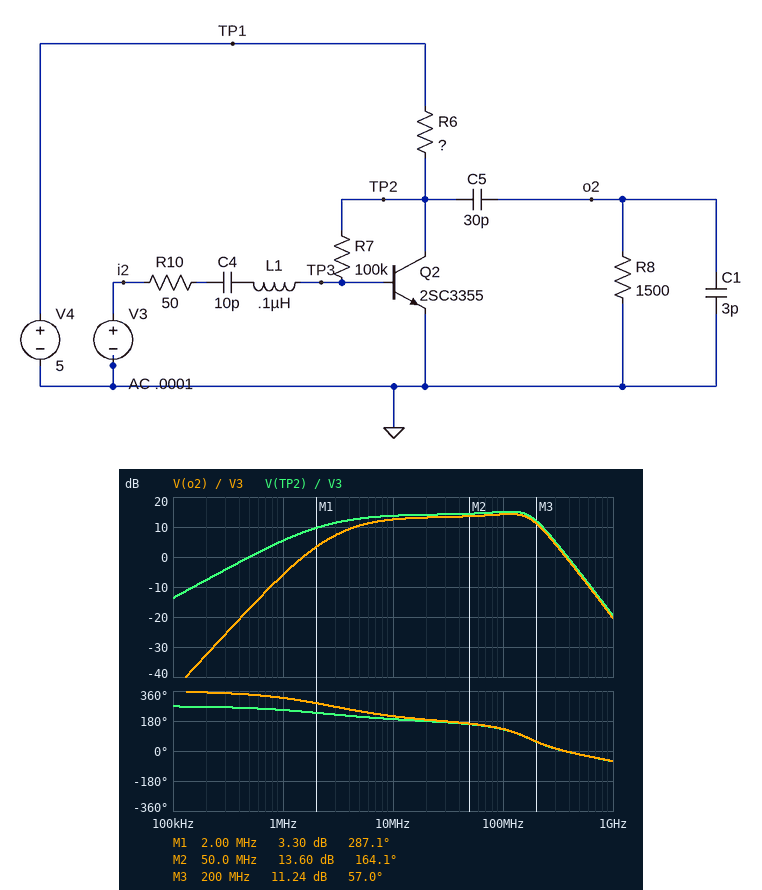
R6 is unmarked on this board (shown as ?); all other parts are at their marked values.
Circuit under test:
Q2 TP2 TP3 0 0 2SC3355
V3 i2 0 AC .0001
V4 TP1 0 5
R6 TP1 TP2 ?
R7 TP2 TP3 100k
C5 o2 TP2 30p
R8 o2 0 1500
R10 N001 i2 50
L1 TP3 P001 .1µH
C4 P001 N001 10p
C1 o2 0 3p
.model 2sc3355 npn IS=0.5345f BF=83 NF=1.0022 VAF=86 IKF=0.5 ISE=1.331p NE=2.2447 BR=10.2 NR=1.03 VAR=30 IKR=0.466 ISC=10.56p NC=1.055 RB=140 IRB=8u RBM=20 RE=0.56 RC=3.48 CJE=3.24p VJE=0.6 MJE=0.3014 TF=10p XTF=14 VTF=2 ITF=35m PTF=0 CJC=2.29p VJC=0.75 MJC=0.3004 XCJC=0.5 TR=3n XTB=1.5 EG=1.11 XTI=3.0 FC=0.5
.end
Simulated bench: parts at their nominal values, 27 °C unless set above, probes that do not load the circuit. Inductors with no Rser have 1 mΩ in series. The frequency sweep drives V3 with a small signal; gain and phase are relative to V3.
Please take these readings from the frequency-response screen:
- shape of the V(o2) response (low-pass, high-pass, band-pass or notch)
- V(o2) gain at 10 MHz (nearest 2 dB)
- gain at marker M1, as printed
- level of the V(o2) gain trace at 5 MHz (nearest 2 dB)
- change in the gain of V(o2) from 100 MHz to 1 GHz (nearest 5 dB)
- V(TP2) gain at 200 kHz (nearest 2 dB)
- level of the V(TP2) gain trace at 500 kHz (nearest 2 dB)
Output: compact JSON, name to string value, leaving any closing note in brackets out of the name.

{"shape of the V(o2) response": "band-pass", "V(o2) gain at 10 MHz": "12 dB", "gain at marker M1, as printed": "3.30 dB", "level of the V(o2) gain trace at 5 MHz": "10 dB", "change in the gain of V(o2) from 100 MHz to 1 GHz": "-35 dB", "V(TP2) gain at 200 kHz": "-8 dB", "level of the V(TP2) gain trace at 500 kHz": "0 dB"}
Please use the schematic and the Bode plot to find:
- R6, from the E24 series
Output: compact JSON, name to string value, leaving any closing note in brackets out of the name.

{"R6, from the E24 series": "620 Ω"}
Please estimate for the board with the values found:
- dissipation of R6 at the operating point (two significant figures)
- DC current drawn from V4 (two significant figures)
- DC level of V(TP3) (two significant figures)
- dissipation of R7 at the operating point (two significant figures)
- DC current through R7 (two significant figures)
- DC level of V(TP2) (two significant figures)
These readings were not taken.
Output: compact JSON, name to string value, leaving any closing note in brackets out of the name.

{"dissipation of R6 at the operating point": "3.3 mW", "DC current drawn from V4": "2.3 mA", "DC level of V(TP3)": "760 mV", "dissipation of R7 at the operating point": "79 µW", "DC current through R7": "28 µA", "DC level of V(TP2)": "3.6 V"}
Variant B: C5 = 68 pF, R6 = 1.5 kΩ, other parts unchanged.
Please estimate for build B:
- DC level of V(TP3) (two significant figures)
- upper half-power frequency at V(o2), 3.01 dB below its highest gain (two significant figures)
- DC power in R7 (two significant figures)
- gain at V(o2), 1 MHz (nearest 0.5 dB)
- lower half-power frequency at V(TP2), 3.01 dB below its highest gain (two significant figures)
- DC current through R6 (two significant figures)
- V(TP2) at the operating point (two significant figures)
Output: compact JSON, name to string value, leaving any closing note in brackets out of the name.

{"DC level of V(TP3)": "750 mV", "upper half-power frequency at V(o2), 3.01 dB below its highest gain": "190 MHz", "DC power in R7": "37 µW", "gain at V(o2), 1 MHz": "2.5 dB", "lower half-power frequency at V(TP2), 3.01 dB below its highest gain": "2.1 MHz", "DC current through R6": "1.6 mA", "V(TP2) at the operating point": "2.7 V"}
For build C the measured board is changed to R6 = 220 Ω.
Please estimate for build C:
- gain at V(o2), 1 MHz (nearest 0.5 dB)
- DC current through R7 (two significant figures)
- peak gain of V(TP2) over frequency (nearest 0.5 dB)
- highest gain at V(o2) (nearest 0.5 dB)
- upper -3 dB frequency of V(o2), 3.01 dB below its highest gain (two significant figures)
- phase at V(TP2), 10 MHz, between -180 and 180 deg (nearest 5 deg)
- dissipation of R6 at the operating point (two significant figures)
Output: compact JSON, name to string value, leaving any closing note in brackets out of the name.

{"gain at V(o2), 1 MHz": "-12.0 dB", "DC current through R7": "36 µA", "peak gain of V(TP2) over frequency": "14.5 dB", "highest gain at V(o2)": "14.0 dB", "upper -3 dB frequency of V(o2), 3.01 dB below its highest gain": "210 MHz", "phase at V(TP2), 10 MHz, between -180 and 180 deg": "-160 deg", "dissipation of R6 at the operating point": "2.0 mW"}
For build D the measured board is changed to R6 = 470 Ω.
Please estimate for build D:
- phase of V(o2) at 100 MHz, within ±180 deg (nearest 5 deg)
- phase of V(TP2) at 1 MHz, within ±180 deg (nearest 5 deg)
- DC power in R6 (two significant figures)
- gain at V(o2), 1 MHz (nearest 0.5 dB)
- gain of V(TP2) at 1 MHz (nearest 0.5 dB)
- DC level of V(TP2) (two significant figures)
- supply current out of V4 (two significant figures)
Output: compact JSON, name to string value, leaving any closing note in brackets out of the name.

{"phase of V(o2) at 100 MHz, within ±180 deg": "135 deg", "phase of V(TP2) at 1 MHz, within ±180 deg": "-110 deg", "DC power in R6": "3.0 mW", "gain at V(o2), 1 MHz": "-7.5 dB", "gain of V(TP2) at 1 MHz": "4.0 dB", "DC level of V(TP2)": "3.8 V", "supply current out of V4": "2.5 mA"}
